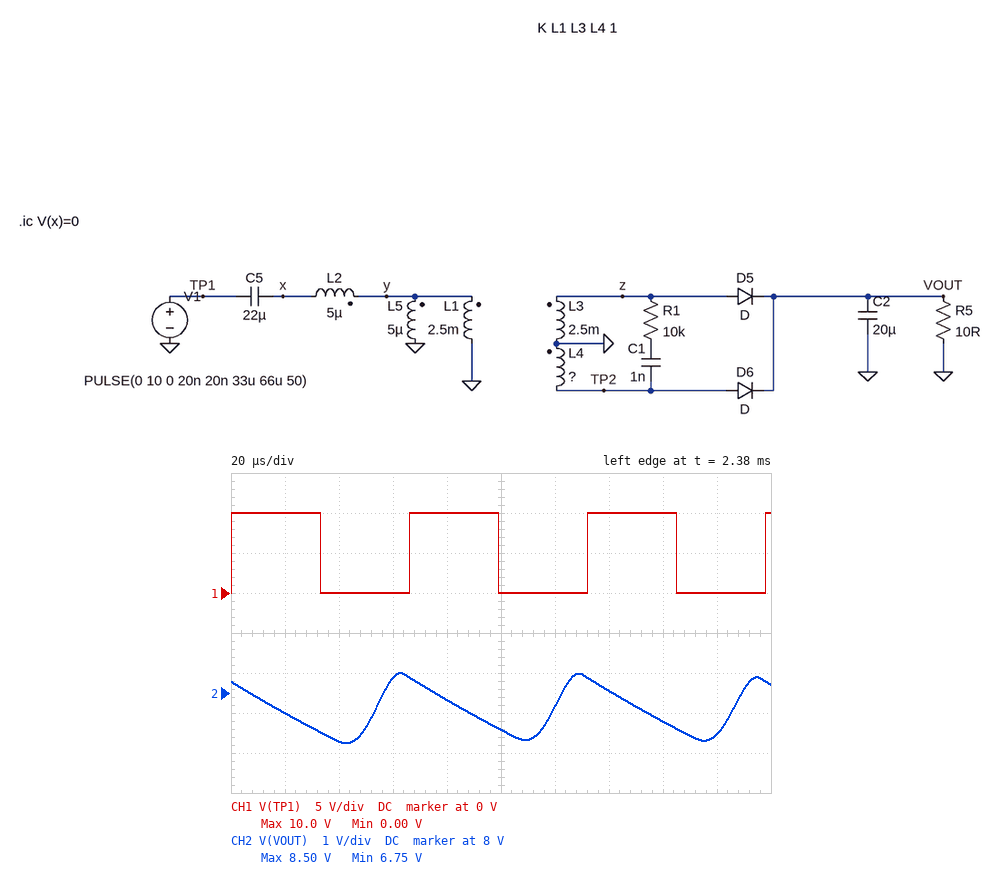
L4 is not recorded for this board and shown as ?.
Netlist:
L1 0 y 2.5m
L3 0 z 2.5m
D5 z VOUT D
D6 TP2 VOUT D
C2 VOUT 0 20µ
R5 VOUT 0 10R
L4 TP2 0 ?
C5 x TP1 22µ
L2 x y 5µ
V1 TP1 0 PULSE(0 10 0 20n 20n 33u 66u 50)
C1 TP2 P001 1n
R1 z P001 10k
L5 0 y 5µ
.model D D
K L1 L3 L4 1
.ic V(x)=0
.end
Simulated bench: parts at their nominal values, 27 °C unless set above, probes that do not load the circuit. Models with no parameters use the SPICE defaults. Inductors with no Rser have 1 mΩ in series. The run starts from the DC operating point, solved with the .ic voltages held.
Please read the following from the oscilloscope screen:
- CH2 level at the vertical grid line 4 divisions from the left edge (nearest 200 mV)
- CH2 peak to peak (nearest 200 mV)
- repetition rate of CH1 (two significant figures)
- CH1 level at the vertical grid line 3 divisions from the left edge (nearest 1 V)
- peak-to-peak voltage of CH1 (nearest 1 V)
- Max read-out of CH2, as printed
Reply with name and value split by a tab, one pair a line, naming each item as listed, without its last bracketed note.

CH2 level at the vertical grid line 4 divisions from the left edge	7.8 V
CH2 peak to peak	1.8 V
repetition rate of CH1	15 kHz
CH1 level at the vertical grid line 3 divisions from the left edge	0 V
peak-to-peak voltage of CH1	10 V
Max read-out of CH2, as printed	8.50 V
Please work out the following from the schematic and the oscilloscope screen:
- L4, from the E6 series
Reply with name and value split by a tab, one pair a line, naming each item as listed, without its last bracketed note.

L4, from the E6 series	6.8 mH
